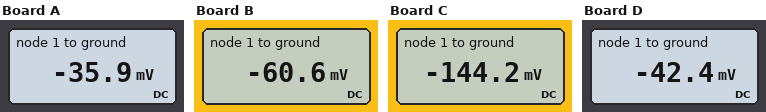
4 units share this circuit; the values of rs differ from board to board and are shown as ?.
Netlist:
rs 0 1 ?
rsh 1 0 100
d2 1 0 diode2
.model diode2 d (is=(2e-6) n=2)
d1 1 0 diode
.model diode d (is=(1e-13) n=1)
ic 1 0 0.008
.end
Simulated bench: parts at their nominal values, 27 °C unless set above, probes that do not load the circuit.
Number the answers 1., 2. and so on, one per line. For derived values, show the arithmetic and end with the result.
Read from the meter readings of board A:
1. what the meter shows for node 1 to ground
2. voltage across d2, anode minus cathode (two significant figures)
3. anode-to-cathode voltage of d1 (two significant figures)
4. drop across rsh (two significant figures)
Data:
1. -35.9 mV
2. -35.9 mV = -36 mV
3. -35.9 mV = -36 mV
4. 0 V - (-35.9 mV) = 36 mV
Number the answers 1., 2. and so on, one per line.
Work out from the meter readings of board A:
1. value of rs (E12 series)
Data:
1. 4.7 Ω
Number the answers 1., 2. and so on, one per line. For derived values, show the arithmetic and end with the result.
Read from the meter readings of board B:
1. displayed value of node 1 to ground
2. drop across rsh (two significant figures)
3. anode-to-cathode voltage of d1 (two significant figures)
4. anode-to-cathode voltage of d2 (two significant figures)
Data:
1. -60.6 mV
2. 0 V - (-60.6 mV) = 61 mV
3. -60.6 mV = -61 mV
4. -60.6 mV = -61 mV
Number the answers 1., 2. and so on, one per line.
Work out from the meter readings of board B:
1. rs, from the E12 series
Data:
1. 8.2 Ω
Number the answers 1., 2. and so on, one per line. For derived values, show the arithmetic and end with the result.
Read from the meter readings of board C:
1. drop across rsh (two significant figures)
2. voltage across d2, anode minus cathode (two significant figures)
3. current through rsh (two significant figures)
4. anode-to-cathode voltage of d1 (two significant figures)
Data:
1. 0 V - (-144.2 mV) = 140 mV
2. -144.2 mV = -140 mV
3. (0 V - (-144.2 mV)) / 100 Ω = 1.4 mA
4. -144.2 mV = -140 mV
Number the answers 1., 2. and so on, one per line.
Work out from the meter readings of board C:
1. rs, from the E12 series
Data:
1. 22 Ω
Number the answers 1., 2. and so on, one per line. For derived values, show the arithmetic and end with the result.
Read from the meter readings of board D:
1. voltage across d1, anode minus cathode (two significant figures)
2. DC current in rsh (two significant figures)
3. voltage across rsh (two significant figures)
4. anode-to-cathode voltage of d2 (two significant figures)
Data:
1. -42.4 mV = -42 mV
2. (0 V - (-42.4 mV)) / 100 Ω = 420 µA
3. 0 V - (-42.4 mV) = 42 mV
4. -42.4 mV = -42 mV
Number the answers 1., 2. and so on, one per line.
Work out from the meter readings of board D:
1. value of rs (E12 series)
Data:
1. 5.6 Ω
